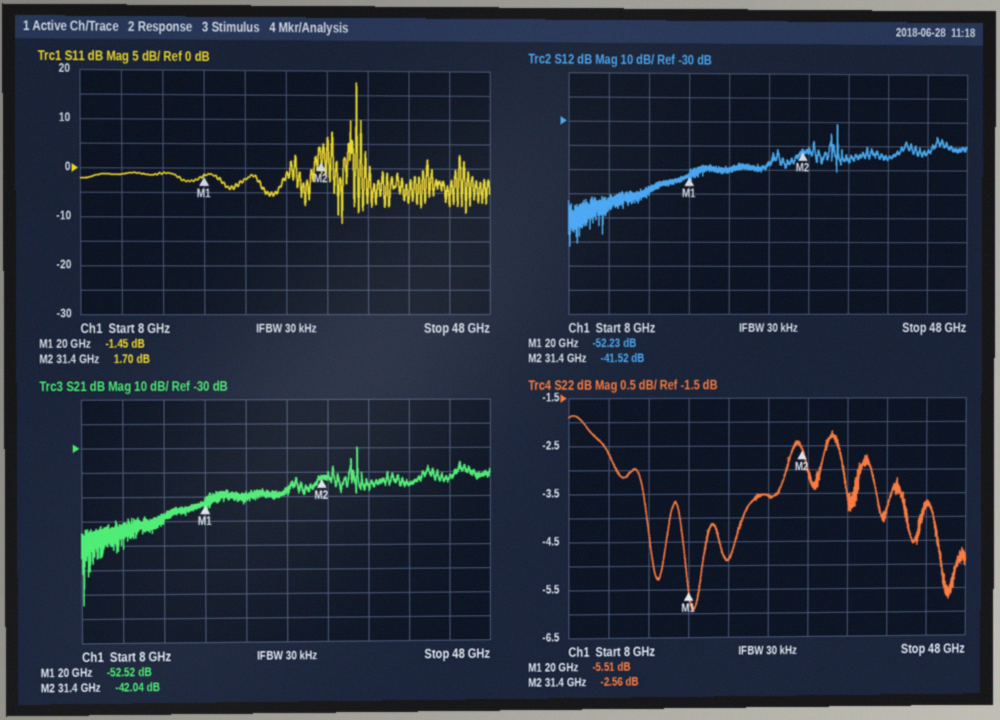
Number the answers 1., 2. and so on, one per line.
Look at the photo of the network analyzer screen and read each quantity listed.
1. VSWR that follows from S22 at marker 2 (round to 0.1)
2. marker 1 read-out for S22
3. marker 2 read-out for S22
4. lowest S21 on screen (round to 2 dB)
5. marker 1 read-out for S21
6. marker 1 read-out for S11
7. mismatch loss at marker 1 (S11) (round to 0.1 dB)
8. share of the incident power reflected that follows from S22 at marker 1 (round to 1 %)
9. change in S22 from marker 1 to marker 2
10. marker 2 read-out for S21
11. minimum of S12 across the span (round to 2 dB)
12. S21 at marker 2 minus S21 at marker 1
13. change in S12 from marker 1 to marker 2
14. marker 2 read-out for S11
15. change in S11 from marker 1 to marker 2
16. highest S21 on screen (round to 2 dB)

1. 6.8
2. -5.51 dB
3. -2.56 dB
4. -94 dB
5. -52.52 dB
6. -1.45 dB
7. 5.5 dB
8. 28 %
9. 2.95 dB
10. -42.04 dB
11. -82 dB
12. 10.48 dB
13. 10.71 dB
14. 1.70 dB
15. 3.15 dB
16. -30 dB
